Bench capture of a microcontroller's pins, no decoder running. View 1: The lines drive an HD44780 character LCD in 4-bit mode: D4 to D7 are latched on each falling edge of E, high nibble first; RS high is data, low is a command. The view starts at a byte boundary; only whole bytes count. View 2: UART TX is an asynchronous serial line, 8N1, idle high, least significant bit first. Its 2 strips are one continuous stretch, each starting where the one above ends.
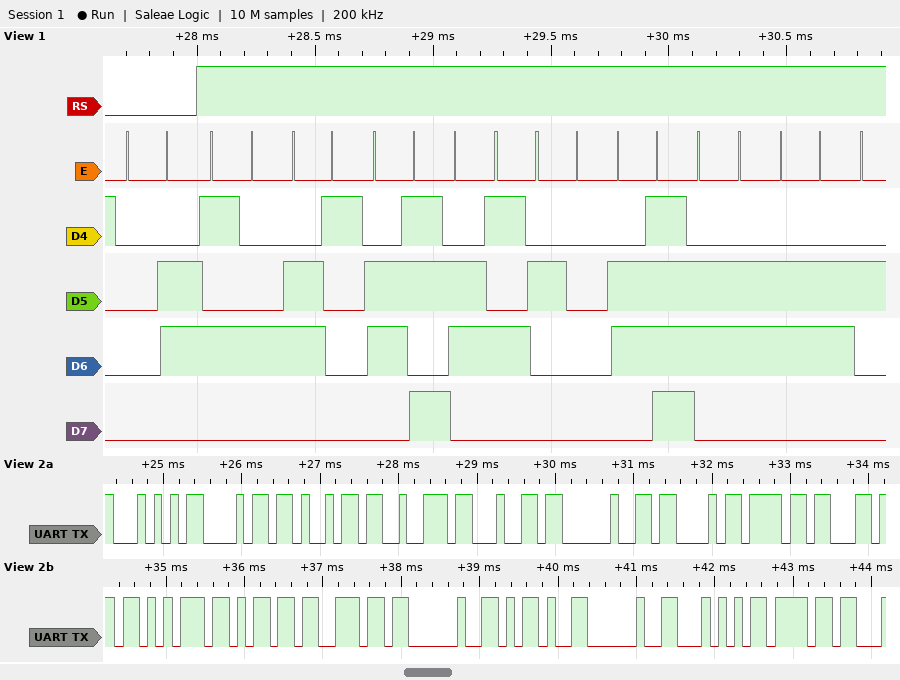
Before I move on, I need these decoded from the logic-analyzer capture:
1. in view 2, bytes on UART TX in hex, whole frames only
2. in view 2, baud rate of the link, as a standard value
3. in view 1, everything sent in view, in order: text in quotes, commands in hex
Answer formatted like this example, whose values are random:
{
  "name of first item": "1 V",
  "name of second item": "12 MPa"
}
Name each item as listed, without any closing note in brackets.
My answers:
{
  "in view 2, bytes on UART TX in hex, whole frames only": "0x54 0x68 0x69 0x72 0x64 0x20 0x43 0x6F 0x6C 0x75 0x6D 0x6E 0x20 0x2D 0x20 0x54 0x6F",
  "in view 2, baud rate of the link, as a standard value": "9600 baud",
  "in view 1, everything sent in view, in order: text in quotes, commands in hex": "0x06 \"Take off\""
}
